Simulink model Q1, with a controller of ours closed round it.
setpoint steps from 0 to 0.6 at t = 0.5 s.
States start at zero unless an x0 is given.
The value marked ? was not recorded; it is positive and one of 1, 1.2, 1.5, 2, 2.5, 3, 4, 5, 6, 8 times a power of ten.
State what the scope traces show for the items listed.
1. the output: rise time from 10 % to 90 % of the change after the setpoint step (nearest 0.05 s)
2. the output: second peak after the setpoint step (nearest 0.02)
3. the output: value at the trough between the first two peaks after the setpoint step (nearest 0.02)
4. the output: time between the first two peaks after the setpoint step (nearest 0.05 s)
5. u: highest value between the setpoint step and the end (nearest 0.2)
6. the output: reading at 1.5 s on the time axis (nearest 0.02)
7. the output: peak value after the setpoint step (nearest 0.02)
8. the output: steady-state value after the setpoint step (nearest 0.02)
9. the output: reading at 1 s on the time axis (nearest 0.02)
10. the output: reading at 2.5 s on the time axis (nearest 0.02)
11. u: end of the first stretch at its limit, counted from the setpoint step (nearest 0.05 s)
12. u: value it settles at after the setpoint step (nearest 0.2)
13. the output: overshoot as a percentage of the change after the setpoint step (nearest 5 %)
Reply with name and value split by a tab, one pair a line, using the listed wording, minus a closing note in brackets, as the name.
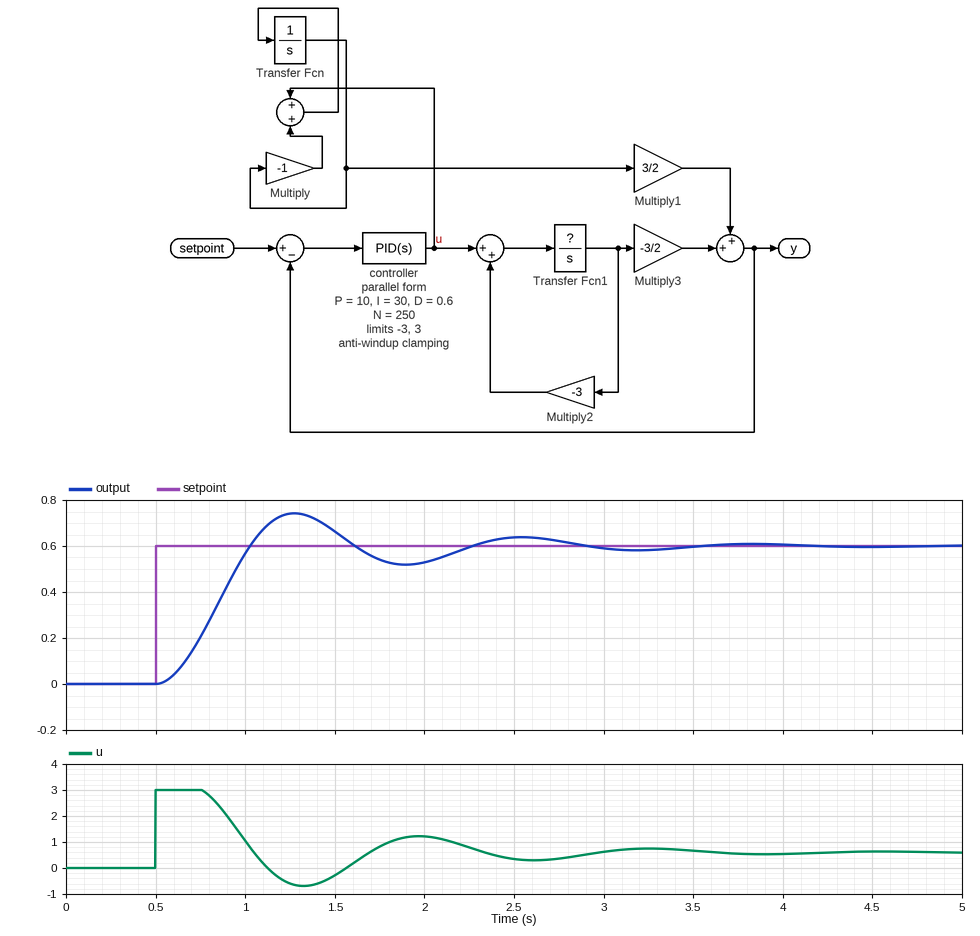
the output: rise time from 10 % to 90 % of the change after the setpoint step	0.35 s
the output: second peak after the setpoint step	0.64
the output: value at the trough between the first two peaks after the setpoint step	0.52
the output: time between the first two peaks after the setpoint step	1.25 s
u: highest value between the setpoint step and the end	3.0
the output: reading at 1.5 s on the time axis	0.66
the output: peak value after the setpoint step	0.74
the output: steady-state value after the setpoint step	0.60
the output: reading at 1 s on the time axis	0.56
the output: reading at 2.5 s on the time axis	0.64
u: end of the first stretch at its limit, counted from the setpoint step	0.25 s
u: value it settles at after the setpoint step	0.6
the output: overshoot as a percentage of the change after the setpoint step	25 %
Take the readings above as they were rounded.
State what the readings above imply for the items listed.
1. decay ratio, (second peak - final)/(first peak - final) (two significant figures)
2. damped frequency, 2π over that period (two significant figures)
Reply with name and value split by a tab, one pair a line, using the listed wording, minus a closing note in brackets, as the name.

decay ratio, (second peak - final)/(first peak - final)	0.29
damped frequency, 2π over that period	5.0 rad/s
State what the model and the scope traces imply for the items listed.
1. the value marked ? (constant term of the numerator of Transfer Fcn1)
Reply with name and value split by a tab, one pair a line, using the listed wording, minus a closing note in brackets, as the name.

the value marked ?	1
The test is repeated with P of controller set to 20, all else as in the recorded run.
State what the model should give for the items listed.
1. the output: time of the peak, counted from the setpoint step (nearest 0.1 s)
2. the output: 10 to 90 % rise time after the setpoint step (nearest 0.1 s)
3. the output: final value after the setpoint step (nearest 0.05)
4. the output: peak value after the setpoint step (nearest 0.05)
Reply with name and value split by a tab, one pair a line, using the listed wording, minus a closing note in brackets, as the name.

the output: time of the peak, counted from the setpoint step	0.7 s
the output: 10 to 90 % rise time after the setpoint step	0.3 s
the output: final value after the setpoint step	0.60
the output: peak value after the setpoint step	0.70
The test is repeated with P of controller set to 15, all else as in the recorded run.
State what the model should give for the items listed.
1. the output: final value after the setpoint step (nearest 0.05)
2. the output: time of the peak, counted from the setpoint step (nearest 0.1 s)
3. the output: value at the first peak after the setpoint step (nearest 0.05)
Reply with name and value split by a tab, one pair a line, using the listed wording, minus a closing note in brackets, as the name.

the output: final value after the setpoint step	0.60
the output: time of the peak, counted from the setpoint step	0.7 s
the output: value at the first peak after the setpoint step	0.70
